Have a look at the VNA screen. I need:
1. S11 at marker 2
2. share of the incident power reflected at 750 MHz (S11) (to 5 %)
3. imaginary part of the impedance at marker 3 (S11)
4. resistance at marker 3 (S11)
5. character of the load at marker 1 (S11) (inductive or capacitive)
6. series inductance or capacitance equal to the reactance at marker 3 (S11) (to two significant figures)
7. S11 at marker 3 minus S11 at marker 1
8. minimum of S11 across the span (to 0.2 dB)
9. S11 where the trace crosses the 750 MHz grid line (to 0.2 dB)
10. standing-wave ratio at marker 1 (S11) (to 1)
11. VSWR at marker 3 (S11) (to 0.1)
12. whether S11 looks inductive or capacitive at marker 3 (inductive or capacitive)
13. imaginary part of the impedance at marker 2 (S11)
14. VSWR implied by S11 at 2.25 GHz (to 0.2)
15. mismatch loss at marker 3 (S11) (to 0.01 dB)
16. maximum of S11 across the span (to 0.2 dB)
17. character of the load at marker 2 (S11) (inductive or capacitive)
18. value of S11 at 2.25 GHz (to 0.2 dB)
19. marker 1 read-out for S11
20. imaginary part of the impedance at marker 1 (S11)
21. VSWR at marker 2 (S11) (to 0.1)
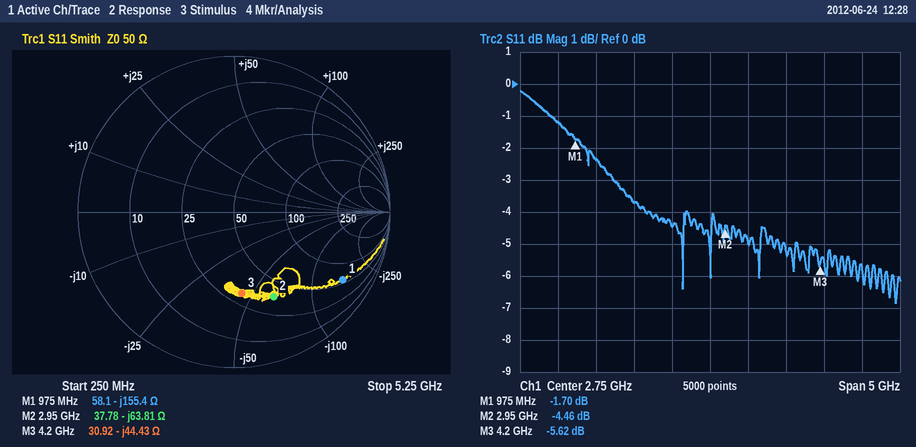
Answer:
-4.46 dB
75 %
-44.43 Ω
30.92 Ω
capacitive
850 fF
-3.92 dB
-6.8 dB
-1.2 dB
10
3.2
capacitive
-63.81 Ω
4.0
1.39 dB
-0.2 dB
capacitive
-4.4 dB
-1.70 dB
-155.4 Ω
4.0
